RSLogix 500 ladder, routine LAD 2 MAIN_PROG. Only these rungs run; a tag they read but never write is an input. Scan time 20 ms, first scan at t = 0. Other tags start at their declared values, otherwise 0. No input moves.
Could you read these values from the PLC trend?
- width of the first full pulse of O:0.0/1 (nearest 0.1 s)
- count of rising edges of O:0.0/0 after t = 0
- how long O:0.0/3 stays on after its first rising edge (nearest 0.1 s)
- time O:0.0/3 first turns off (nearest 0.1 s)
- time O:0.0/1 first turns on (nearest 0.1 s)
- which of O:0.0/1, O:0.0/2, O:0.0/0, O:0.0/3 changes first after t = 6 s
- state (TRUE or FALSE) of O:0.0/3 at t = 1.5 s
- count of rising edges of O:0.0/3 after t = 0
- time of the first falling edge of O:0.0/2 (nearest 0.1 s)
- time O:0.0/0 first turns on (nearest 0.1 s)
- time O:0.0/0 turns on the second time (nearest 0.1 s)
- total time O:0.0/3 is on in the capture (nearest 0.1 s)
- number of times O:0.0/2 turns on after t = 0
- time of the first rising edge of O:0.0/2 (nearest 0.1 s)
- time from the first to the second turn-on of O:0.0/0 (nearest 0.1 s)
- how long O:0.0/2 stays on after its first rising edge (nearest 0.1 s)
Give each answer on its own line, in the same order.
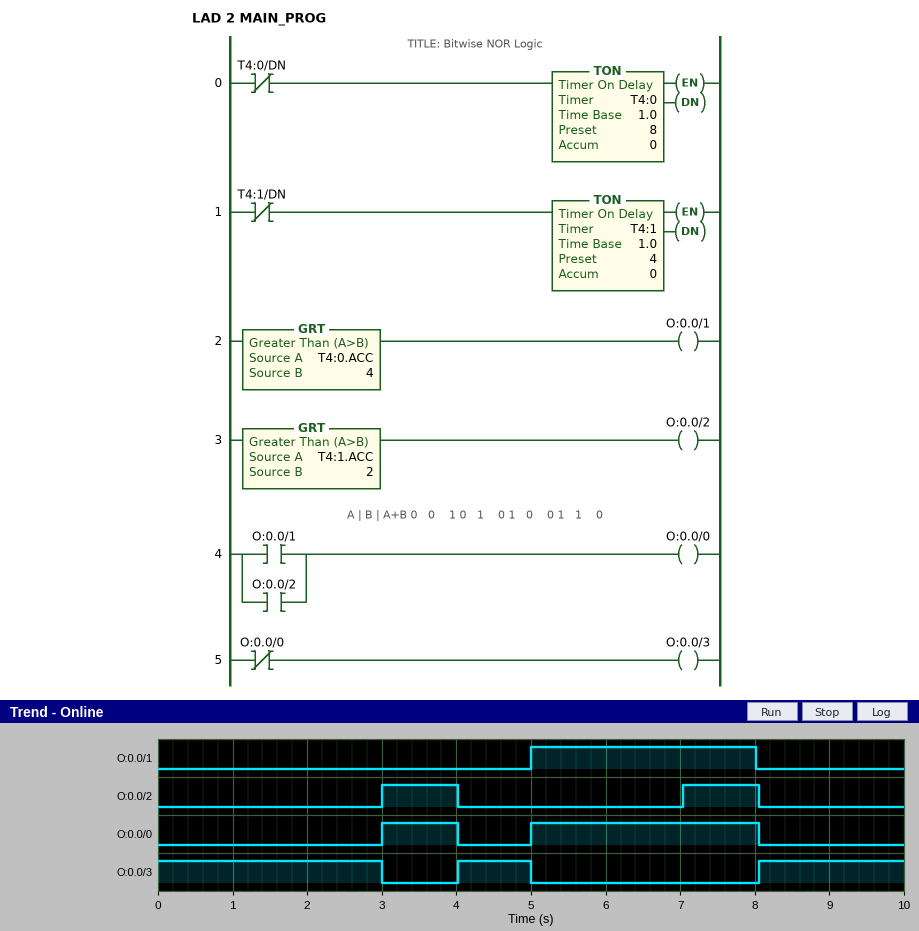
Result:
3.0 s
2
1.0 s
3.0 s
5.0 s
O:0.0/2
TRUE
2
4.0 s
3.0 s
5.0 s
5.9 s
2
3.0 s
2.0 s
1.0 s
